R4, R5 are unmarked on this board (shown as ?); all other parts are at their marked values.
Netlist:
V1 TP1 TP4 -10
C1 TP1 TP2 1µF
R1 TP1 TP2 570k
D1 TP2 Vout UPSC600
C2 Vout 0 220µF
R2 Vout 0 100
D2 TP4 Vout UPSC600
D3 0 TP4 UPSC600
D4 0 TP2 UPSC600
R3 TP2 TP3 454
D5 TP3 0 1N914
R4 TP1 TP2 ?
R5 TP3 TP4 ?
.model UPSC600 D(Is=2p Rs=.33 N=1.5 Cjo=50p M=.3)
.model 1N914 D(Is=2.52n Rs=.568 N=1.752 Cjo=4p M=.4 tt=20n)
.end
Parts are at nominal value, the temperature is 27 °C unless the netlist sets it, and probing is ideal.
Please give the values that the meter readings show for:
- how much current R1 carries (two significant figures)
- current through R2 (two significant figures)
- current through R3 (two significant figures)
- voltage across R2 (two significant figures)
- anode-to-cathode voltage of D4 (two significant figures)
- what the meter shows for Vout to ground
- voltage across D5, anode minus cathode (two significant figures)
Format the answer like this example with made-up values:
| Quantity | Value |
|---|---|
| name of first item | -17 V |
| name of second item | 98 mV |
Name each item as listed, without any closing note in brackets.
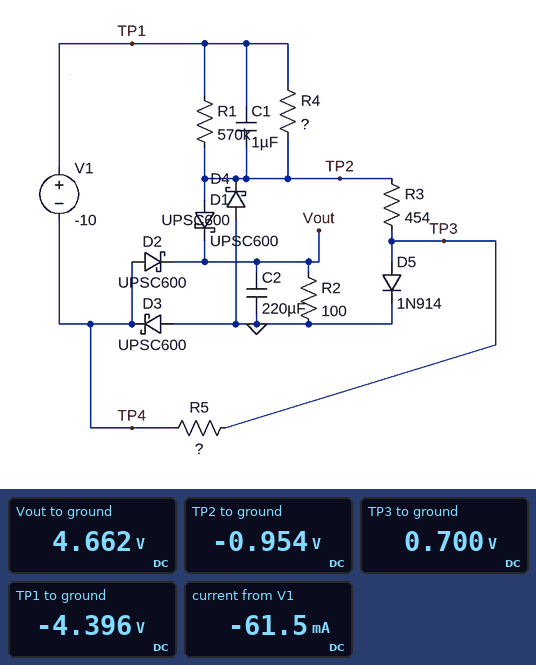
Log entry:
| Quantity | Value |
|---|---|
| how much current R1 carries | 6.0 µA |
| current through R2 | 47 mA |
| current through R3 | 3.6 mA |
| voltage across R2 | 4.7 V |
| anode-to-cathode voltage of D4 | 950 mV |
| what the meter shows for Vout to ground | 4.662 V |
| voltage across D5, anode minus cathode | 700 mV |
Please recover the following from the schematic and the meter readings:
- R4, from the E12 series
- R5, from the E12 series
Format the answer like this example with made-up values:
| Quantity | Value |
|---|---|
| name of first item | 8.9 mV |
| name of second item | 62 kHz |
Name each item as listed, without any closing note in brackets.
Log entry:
| Quantity | Value |
|---|---|
| R4, from the E12 series | 56 Ω |
| R5, from the E12 series | 330 Ω |
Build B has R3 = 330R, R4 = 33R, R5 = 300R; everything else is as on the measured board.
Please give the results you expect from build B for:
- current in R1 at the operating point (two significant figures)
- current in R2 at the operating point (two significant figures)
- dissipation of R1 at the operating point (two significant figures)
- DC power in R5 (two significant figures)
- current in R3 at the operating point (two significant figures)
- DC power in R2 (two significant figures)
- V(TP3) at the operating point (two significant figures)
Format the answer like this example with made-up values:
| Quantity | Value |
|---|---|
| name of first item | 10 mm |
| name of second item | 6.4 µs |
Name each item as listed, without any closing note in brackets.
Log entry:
| Quantity | Value |
|---|---|
| current in R1 at the operating point | 4.4 µA |
| current in R2 at the operating point | 56 mA |
| dissipation of R1 at the operating point | 11 µW |
| DC power in R5 | 110 mW |
| current in R3 at the operating point | 5.1 mA |
| DC power in R2 | 310 mW |
| V(TP3) at the operating point | 710 mV |
